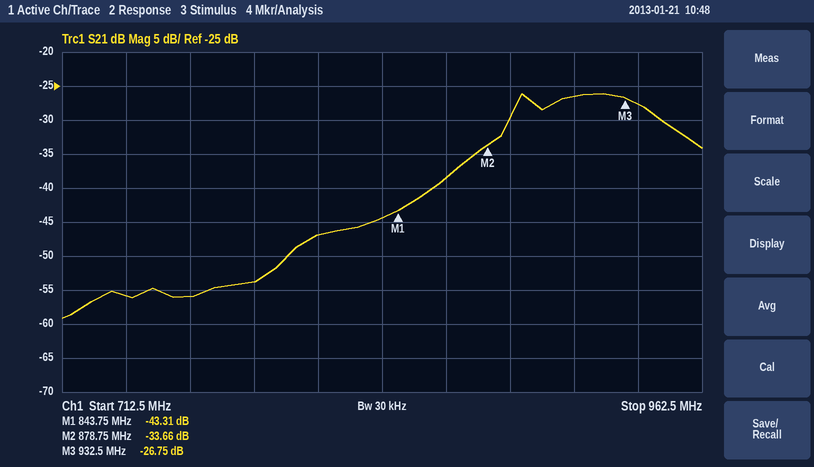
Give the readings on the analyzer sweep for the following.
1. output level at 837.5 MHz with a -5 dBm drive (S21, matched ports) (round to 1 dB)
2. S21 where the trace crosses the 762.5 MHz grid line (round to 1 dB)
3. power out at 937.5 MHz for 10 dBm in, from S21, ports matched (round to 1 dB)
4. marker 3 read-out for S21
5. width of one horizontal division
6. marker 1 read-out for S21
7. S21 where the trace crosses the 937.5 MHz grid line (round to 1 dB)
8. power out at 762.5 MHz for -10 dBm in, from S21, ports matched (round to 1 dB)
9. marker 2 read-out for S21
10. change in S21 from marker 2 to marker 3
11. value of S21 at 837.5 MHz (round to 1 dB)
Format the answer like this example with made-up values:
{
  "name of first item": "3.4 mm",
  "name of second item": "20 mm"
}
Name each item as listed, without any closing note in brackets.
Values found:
{
  "output level at 837.5 MHz with a -5 dBm drive (S21, matched ports)": "-49 dBm",
  "S21 where the trace crosses the 762.5 MHz grid line": "-56 dB",
  "power out at 937.5 MHz for 10 dBm in, from S21, ports matched": "-18 dBm",
  "marker 3 read-out for S21": "-26.75 dB",
  "width of one horizontal division": "25 MHz",
  "marker 1 read-out for S21": "-43.31 dB",
  "S21 where the trace crosses the 937.5 MHz grid line": "-28 dB",
  "power out at 762.5 MHz for -10 dBm in, from S21, ports matched": "-66 dBm",
  "marker 2 read-out for S21": "-33.66 dB",
  "change in S21 from marker 2 to marker 3": "6.91 dB",
  "value of S21 at 837.5 MHz": "-44 dB"
}
